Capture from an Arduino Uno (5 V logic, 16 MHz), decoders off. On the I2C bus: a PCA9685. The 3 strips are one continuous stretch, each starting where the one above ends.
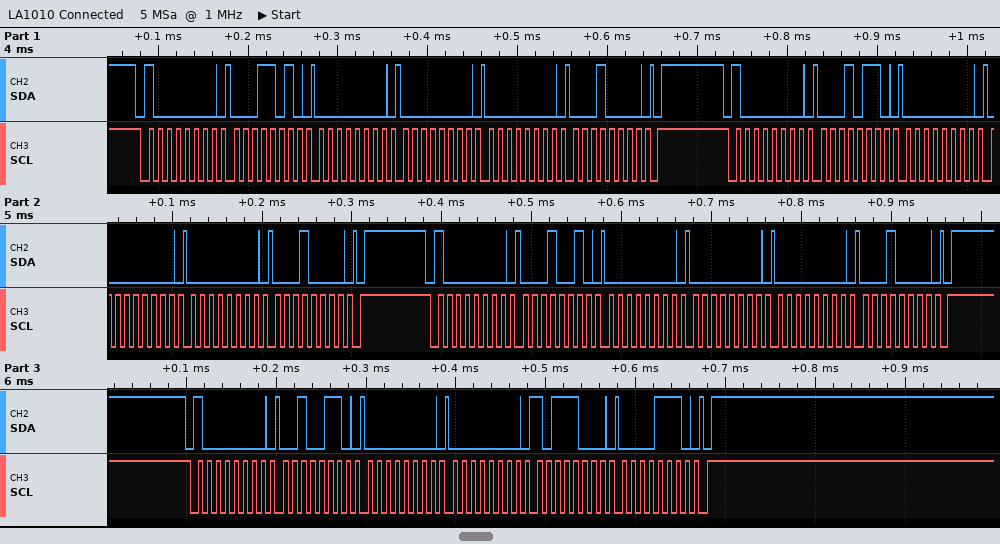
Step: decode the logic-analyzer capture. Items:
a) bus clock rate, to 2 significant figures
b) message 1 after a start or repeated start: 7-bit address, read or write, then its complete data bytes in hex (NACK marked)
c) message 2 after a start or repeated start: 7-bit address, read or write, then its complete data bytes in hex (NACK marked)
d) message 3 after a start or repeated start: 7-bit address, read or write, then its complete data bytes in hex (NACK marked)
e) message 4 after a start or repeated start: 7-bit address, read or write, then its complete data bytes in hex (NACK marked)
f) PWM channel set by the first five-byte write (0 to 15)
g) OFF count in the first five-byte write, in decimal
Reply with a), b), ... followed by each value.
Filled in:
a) 100 kHz
b) 0x40 write: 1A 00 00 00 10
c) 0x40 write: 16 00 00 00 10
d) 0x40 write: 12 00 00 00 10
e) 0x40 write: 26 00 00 B8 0E
f) 5
g) 4096
